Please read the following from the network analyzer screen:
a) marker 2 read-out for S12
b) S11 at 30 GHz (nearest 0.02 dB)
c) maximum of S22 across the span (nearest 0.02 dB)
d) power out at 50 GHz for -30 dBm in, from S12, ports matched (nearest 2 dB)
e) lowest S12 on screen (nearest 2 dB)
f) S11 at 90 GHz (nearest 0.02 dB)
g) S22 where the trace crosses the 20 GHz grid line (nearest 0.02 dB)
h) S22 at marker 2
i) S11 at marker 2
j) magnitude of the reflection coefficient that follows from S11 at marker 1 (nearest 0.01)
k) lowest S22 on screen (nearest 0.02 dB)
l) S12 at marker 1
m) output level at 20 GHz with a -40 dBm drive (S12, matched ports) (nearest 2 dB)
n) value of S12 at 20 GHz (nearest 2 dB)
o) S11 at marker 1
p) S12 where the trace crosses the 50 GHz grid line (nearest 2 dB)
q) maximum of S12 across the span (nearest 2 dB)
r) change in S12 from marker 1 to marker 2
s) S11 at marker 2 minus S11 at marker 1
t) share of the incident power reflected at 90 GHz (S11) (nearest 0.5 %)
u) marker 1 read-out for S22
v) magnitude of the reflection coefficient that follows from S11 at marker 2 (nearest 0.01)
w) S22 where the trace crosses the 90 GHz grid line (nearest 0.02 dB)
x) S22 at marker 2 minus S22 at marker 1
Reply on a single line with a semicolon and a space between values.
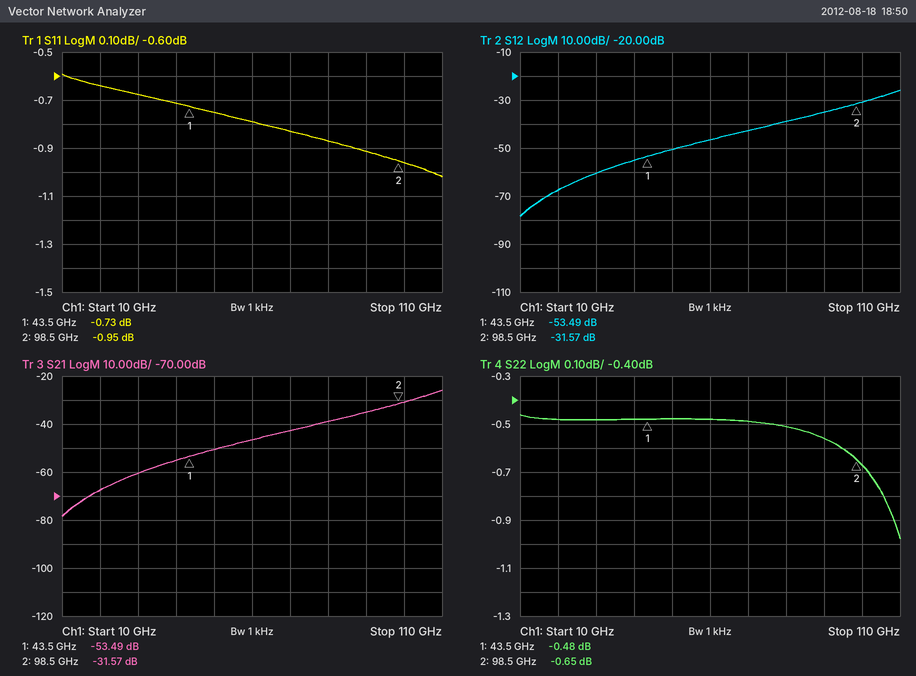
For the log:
-31.57 dB; -0.68 dB; -0.46 dB; -80 dBm; -78 dB; -0.92 dB; -0.48 dB; -0.65 dB; -0.95 dB; 0.92; -0.98 dB; -53.49 dB; -108 dBm; -68 dB; -0.73 dB; -50 dB; -26 dB; 21.92 dB; -0.22 dB; 81.0 %; -0.48 dB; 0.90; -0.56 dB; -0.17 dB
